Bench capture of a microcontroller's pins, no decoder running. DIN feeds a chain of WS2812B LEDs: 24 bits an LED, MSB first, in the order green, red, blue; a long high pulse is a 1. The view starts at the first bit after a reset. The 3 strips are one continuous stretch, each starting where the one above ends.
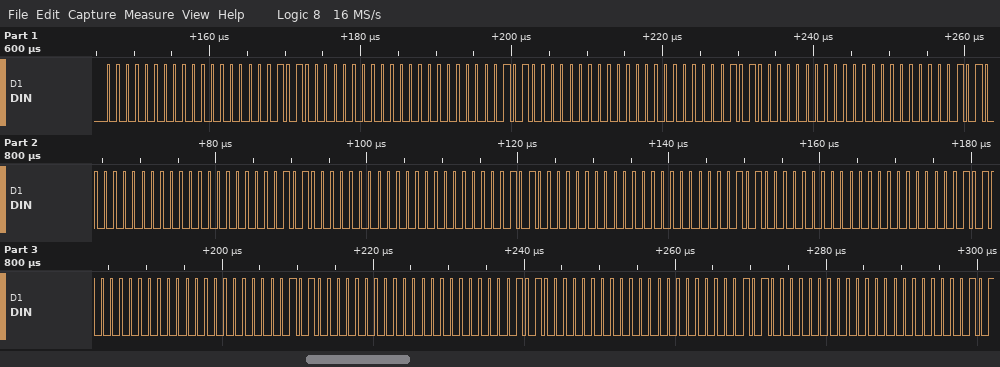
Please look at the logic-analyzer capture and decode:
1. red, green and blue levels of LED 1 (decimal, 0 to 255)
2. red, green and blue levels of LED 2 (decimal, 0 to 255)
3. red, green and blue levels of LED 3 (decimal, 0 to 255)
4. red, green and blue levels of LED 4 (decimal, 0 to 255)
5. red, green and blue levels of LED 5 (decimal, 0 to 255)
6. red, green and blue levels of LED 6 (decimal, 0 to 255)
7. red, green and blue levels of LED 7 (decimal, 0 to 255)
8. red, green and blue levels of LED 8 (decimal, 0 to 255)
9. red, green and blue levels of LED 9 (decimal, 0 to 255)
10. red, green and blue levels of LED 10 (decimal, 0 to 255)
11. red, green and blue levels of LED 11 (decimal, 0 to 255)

0, 0, 40
0, 0, 40
0, 0, 40
0, 0, 40
0, 0, 40
0, 0, 40
0, 0, 40
0, 0, 40
0, 0, 40
0, 0, 40
0, 0, 40
